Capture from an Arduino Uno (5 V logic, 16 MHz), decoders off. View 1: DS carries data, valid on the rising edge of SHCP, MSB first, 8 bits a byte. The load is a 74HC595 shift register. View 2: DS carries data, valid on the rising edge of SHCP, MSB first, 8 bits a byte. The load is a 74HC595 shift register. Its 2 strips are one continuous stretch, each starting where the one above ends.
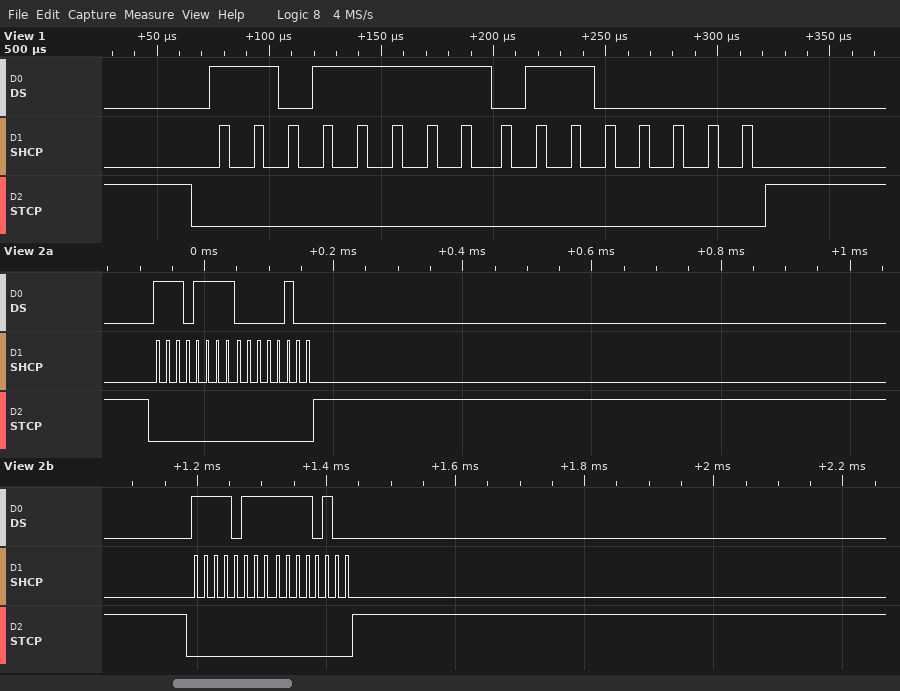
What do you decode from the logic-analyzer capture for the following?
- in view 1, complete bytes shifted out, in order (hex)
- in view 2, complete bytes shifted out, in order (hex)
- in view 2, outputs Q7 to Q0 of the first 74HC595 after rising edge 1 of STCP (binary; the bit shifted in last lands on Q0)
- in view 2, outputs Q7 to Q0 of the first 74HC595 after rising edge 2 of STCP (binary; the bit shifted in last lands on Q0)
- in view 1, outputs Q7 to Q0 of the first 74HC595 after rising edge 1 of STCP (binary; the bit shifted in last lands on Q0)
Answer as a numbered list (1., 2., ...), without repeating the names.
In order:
1. DF 60
2. EF 04 F7 F4
3. 00000100
4. 11110100
5. 01100000
